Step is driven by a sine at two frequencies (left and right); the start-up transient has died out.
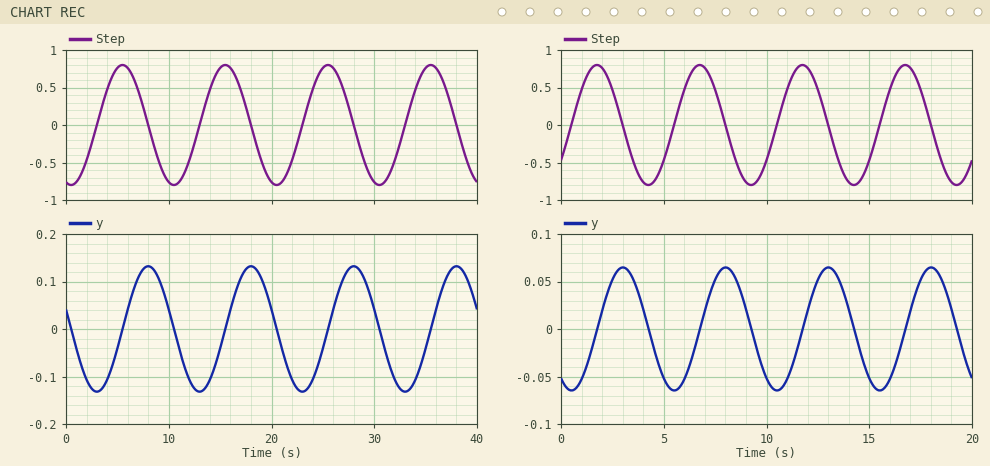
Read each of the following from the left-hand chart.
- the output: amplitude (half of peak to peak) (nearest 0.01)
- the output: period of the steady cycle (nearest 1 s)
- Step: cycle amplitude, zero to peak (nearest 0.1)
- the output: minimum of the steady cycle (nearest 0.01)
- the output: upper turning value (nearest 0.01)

0.13
10 s
0.8
-0.13
0.13
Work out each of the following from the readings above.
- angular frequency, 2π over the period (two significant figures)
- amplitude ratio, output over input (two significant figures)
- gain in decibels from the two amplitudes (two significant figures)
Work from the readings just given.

0.63 rad/s
0.16
-16 dB
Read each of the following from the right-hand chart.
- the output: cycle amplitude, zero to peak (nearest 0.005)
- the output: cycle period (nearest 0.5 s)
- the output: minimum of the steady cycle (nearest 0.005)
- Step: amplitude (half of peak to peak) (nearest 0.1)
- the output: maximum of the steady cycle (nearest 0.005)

0.065
5.0 s
-0.065
0.8
0.065
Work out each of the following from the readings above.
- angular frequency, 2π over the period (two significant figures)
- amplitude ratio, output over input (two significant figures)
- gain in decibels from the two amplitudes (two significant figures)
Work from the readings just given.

1.3 rad/s
0.081
-22 dB
